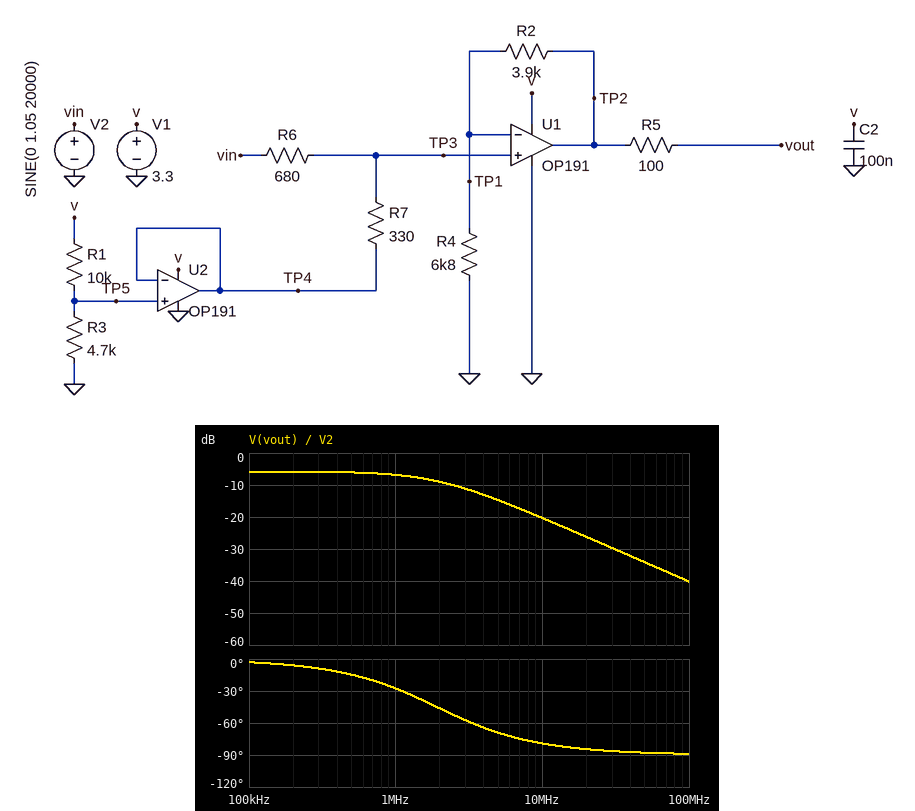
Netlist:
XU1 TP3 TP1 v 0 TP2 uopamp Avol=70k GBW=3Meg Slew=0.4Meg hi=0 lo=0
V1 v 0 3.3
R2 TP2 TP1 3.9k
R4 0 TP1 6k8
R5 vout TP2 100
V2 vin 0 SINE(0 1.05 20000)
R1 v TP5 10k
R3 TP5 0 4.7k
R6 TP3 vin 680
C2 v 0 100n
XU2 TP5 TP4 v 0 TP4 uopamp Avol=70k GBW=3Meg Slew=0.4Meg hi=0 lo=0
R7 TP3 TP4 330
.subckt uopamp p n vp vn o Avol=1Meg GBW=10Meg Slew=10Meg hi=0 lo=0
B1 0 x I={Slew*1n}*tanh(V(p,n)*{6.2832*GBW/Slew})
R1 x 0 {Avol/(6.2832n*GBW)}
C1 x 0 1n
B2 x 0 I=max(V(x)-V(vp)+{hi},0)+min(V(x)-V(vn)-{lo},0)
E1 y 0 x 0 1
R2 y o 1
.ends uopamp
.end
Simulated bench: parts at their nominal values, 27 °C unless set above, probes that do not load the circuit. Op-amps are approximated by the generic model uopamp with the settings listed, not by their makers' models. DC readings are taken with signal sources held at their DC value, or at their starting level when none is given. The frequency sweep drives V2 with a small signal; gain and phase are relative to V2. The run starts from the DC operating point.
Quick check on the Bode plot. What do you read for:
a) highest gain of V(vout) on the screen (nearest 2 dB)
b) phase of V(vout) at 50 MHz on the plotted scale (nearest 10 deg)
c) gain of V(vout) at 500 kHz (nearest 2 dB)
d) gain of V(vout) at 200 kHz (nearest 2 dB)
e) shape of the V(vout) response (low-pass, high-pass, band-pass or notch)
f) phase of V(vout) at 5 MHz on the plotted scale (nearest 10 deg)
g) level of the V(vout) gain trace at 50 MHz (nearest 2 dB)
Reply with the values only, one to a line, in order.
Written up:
-6 dB
-90 deg
-6 dB
-6 dB
low-pass
-70 deg
-34 dB
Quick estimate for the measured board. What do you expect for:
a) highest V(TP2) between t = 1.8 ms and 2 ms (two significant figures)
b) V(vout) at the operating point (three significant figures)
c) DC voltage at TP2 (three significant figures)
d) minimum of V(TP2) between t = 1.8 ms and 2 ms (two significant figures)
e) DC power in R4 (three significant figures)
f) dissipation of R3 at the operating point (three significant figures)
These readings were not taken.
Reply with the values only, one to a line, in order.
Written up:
1.7 V
1.12 V
1.12 V
580 mV
74.2 µW
237 µW
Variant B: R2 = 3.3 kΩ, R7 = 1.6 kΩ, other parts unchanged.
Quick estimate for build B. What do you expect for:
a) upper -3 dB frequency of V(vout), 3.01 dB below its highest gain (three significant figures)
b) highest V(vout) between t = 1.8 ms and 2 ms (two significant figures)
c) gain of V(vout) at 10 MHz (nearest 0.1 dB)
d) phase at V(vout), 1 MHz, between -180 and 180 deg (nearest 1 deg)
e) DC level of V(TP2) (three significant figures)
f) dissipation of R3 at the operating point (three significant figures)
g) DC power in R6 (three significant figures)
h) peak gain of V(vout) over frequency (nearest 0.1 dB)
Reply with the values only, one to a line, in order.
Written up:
2.02 MHz
1.6 V
-13.7 dB
-26 deg
467 mV
237 µW
146 µW
0.4 dB
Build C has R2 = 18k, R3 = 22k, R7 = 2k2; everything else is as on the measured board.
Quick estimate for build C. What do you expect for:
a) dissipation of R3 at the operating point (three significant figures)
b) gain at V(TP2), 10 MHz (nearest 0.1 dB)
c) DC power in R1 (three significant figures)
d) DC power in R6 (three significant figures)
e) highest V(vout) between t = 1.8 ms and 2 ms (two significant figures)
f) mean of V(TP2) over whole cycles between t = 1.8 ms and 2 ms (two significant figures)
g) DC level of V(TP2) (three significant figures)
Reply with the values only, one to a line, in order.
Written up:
234 µW
-12.8 dB
106 µW
422 µW
3.3 V
1.8 V
1.95 V
